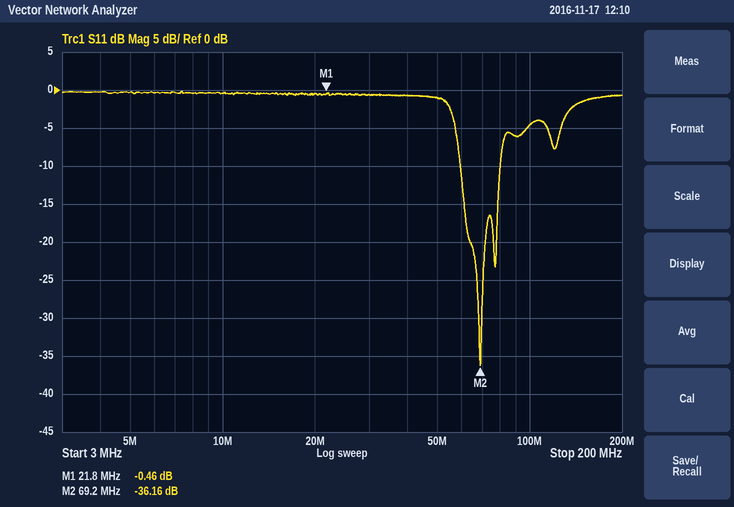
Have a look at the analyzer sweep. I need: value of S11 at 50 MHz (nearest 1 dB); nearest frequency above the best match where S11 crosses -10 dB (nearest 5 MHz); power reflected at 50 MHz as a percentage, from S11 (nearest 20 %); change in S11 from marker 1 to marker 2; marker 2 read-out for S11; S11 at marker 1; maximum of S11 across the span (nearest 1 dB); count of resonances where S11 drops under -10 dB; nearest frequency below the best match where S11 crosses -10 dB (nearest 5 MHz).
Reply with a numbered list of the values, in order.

1. -1 dB
2. 80 MHz
3. 80 %
4. -35.70 dB
5. -36.16 dB
6. -0.46 dB
7. 0 dB
8. 2
9. 60 MHz
